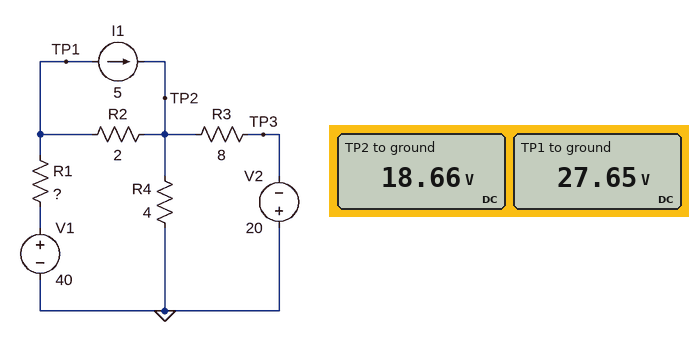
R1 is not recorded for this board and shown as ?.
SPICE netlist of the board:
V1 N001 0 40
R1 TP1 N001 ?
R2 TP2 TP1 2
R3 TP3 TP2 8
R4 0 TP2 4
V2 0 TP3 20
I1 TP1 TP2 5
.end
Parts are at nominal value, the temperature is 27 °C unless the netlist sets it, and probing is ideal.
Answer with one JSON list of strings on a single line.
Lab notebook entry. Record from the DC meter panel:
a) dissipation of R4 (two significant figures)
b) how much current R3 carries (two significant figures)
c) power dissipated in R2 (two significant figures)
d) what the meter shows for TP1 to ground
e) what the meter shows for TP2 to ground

["87 W", "4.8 A", "40 W", "27.65 V", "18.66 V"]
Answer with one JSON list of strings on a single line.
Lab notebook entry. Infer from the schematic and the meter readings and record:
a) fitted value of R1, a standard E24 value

["1.3 Ω"]
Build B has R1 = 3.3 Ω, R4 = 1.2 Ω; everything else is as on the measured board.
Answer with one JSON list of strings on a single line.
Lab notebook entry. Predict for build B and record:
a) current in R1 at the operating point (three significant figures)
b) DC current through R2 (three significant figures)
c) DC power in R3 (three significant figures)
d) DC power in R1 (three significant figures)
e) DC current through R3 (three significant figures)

["8.29 A", "3.29 A", "84.8 W", "227 W", "3.26 A"]
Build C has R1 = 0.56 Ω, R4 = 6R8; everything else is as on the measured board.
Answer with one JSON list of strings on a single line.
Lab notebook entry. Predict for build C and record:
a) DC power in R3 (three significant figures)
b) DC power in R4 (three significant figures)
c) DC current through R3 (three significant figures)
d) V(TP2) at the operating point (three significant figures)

["261 W", "97.1 W", "5.71 A", "25.7 V"]
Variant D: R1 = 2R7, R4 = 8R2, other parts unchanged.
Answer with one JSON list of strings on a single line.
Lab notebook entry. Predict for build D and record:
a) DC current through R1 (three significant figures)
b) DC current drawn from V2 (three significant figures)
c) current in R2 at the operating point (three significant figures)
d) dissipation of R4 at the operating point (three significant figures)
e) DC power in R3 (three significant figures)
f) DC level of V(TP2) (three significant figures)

["6.87 A", "4.71 A", "1.87 A", "38.2 W", "178 W", "17.7 V"]
